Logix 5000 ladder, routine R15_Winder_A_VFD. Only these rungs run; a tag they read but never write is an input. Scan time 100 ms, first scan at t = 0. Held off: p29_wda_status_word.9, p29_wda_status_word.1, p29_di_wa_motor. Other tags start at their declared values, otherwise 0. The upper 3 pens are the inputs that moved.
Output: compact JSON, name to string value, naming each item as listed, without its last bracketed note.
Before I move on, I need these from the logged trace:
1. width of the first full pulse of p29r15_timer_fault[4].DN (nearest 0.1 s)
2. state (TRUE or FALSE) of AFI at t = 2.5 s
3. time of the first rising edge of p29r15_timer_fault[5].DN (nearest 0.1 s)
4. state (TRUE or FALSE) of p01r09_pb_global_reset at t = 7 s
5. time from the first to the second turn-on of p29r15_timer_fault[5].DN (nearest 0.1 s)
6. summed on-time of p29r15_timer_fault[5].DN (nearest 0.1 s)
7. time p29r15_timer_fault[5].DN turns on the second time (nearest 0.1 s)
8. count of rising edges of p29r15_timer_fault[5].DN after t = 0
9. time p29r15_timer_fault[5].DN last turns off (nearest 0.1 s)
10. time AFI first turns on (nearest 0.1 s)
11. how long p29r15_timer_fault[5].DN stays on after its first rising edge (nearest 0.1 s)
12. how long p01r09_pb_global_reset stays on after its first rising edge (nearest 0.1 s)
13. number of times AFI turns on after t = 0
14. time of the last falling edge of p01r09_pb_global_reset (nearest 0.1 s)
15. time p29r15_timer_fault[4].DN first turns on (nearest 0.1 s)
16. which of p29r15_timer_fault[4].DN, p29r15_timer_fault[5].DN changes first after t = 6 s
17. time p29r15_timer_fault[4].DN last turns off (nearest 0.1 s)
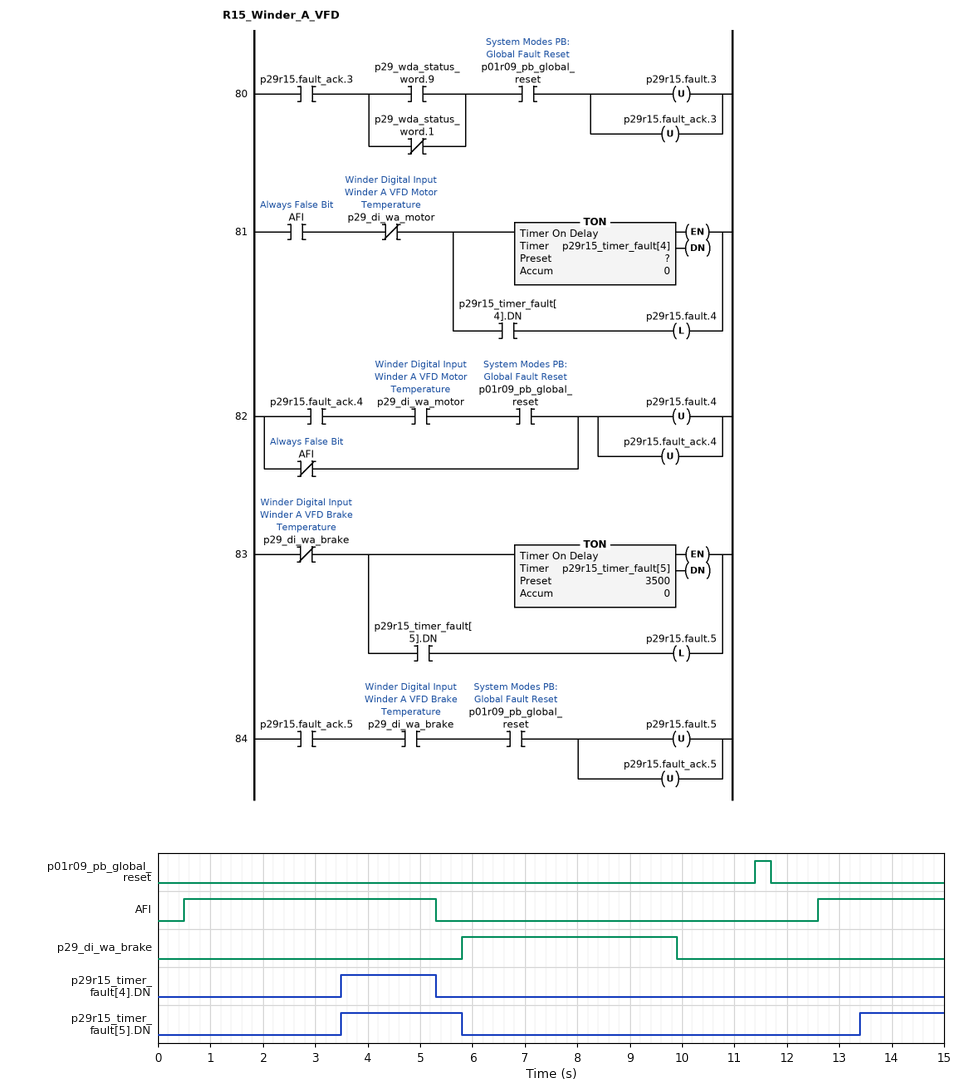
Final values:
{"width of the first full pulse of p29r15_timer_fault[4].DN": "1.8 s", "state (TRUE or FALSE) of AFI at t = 2.5 s": "TRUE", "time of the first rising edge of p29r15_timer_fault[5].DN": "3.5 s", "state (TRUE or FALSE) of p01r09_pb_global_reset at t = 7 s": "FALSE", "time from the first to the second turn-on of p29r15_timer_fault[5].DN": "9.9 s", "summed on-time of p29r15_timer_fault[5].DN": "3.9 s", "time p29r15_timer_fault[5].DN turns on the second time": "13.4 s", "count of rising edges of p29r15_timer_fault[5].DN after t = 0": "2", "time p29r15_timer_fault[5].DN last turns off": "5.8 s", "time AFI first turns on": "0.5 s", "how long p29r15_timer_fault[5].DN stays on after its first rising edge": "2.3 s", "how long p01r09_pb_global_reset stays on after its first rising edge": "0.3 s", "number of times AFI turns on after t = 0": "2", "time of the last falling edge of p01r09_pb_global_reset": "11.7 s", "time p29r15_timer_fault[4].DN first turns on": "3.5 s", "which of p29r15_timer_fault[4].DN, p29r15_timer_fault[5].DN changes first after t = 6 s": "p29r15_timer_fault[5].DN", "time p29r15_timer_fault[4].DN last turns off": "5.3 s"}
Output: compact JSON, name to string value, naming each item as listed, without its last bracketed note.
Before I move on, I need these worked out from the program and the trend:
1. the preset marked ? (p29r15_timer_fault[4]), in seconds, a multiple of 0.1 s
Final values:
{"the preset marked ? (p29r15_timer_fault[4]), in seconds, a multiple of 0.1 s": "3.0 s"}
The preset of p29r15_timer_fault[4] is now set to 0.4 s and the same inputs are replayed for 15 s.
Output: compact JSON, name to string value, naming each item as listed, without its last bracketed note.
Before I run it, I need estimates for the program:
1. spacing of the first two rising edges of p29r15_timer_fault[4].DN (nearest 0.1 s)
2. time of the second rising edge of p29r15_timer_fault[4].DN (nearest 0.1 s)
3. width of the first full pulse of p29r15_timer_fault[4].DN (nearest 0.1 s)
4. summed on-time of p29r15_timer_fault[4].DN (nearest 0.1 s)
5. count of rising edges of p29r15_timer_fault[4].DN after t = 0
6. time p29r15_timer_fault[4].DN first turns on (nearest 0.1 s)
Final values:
{"spacing of the first two rising edges of p29r15_timer_fault[4].DN": "12.1 s", "time of the second rising edge of p29r15_timer_fault[4].DN": "13.0 s", "width of the first full pulse of p29r15_timer_fault[4].DN": "4.4 s", "summed on-time of p29r15_timer_fault[4].DN": "6.4 s", "count of rising edges of p29r15_timer_fault[4].DN after t = 0": "2", "time p29r15_timer_fault[4].DN first turns on": "0.9 s"}
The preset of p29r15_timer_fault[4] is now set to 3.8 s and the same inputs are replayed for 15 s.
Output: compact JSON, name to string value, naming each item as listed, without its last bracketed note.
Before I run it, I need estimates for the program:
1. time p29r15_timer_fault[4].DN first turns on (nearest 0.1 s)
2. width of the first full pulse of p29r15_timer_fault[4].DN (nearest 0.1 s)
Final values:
{"time p29r15_timer_fault[4].DN first turns on": "4.3 s", "width of the first full pulse of p29r15_timer_fault[4].DN": "1.0 s"}
